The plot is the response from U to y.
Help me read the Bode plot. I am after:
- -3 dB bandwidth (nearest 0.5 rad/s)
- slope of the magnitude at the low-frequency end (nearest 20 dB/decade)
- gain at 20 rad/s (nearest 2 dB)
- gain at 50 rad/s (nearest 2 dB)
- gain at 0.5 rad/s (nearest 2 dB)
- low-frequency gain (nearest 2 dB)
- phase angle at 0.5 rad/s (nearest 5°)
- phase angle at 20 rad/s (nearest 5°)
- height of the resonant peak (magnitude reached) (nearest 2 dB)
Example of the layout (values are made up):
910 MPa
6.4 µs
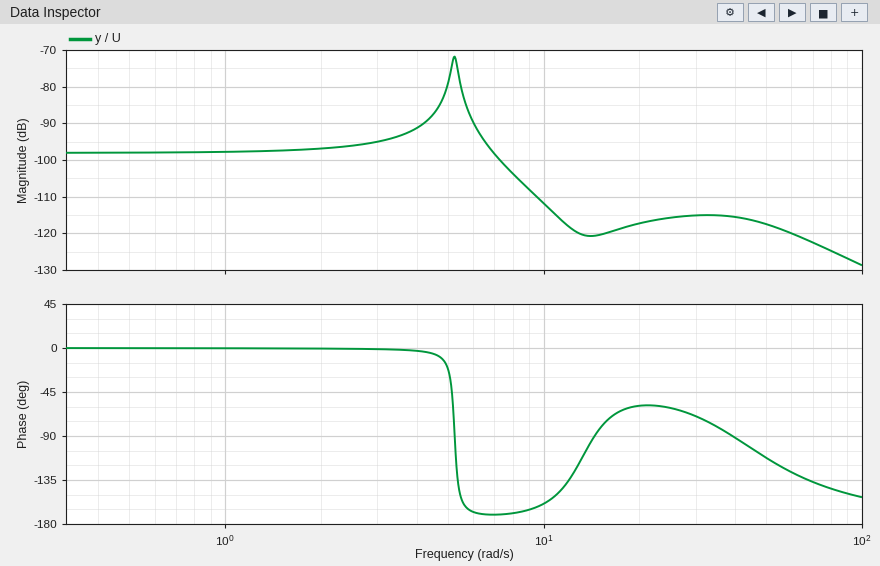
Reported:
7.5 rad/s
0 dB/decade
-118 dB
-118 dB
-98 dB
-98 dB
0°
-60°
-72 dB
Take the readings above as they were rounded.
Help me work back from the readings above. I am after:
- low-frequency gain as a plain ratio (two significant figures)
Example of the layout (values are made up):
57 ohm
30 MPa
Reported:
0.000013
